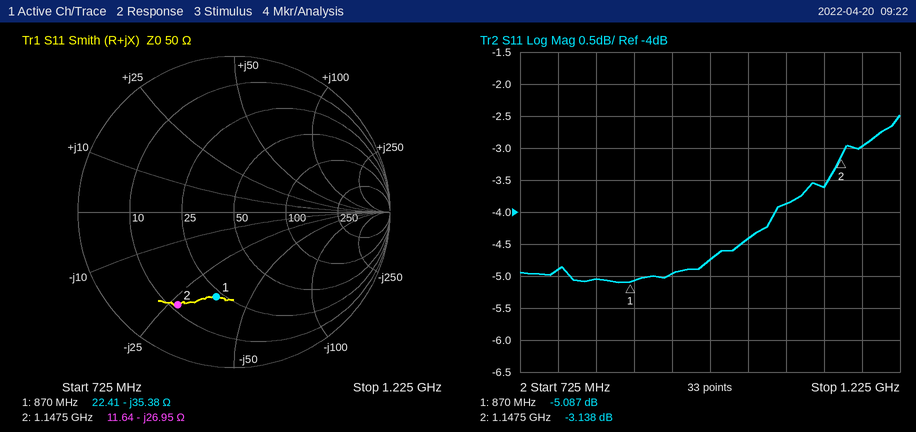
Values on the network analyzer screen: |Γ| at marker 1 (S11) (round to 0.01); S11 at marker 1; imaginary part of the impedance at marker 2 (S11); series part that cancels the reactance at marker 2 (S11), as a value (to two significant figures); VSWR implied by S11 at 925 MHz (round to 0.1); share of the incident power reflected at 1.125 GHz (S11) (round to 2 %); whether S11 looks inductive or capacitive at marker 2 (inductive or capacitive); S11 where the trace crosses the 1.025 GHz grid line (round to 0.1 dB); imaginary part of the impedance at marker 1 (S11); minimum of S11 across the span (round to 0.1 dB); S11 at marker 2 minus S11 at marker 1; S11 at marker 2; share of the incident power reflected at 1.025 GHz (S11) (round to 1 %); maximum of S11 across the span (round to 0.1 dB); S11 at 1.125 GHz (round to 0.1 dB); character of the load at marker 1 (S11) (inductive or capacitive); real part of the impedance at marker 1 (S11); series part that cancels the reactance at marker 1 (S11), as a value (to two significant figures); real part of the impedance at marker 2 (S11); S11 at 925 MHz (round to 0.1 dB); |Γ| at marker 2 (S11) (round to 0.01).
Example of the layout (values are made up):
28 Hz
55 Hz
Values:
0.56
-5.087 dB
-26.95 Ω
3.7 nH
3.6
44 %
capacitive
-4.4 dB
-35.38 Ω
-5.1 dB
1.949 dB
-3.138 dB
36 %
-2.5 dB
-3.6 dB
capacitive
22.41 Ω
6.5 nH
11.64 Ω
-5.0 dB
0.70
